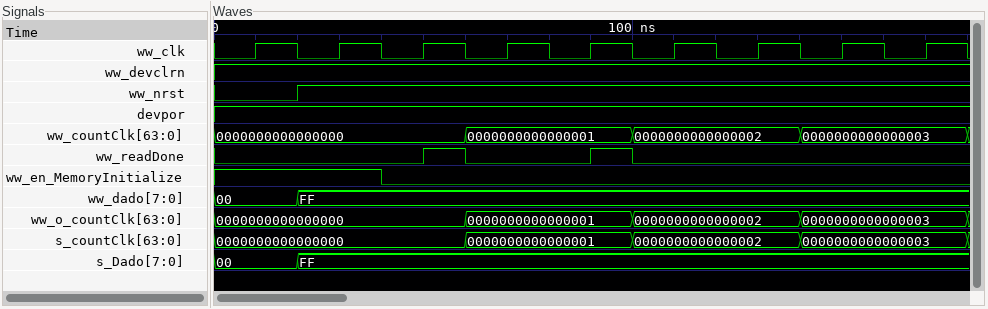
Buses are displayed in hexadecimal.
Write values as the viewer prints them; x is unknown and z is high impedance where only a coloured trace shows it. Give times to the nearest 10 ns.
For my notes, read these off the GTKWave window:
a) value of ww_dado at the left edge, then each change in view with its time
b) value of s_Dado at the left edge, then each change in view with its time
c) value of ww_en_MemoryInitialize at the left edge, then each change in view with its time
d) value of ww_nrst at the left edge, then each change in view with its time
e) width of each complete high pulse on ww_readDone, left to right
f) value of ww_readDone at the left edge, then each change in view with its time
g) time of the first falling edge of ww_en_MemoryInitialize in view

00, FF at 20 ns
00, FF at 20 ns
1, 0 at 40 ns
0, 1 at 20 ns
10 ns, 10 ns
0, 1 at 50 ns, 0 at 60 ns, 1 at 90 ns, 0 at 100 ns
40 ns
